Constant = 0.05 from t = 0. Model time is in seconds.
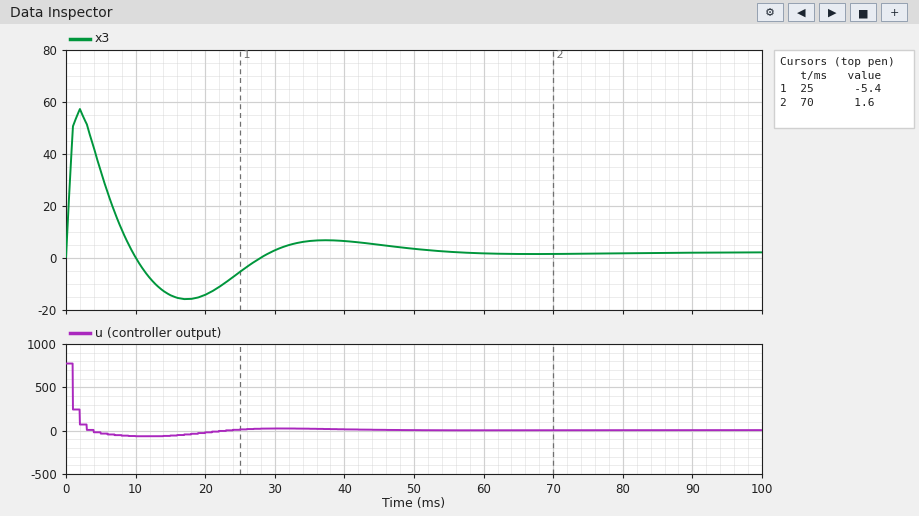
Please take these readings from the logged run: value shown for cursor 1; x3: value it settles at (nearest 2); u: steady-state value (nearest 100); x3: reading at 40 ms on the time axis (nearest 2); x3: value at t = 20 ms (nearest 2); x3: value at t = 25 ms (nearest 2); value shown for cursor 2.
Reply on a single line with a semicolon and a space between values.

-5.4; 2; 0; 6; -14; -6; 1.6
